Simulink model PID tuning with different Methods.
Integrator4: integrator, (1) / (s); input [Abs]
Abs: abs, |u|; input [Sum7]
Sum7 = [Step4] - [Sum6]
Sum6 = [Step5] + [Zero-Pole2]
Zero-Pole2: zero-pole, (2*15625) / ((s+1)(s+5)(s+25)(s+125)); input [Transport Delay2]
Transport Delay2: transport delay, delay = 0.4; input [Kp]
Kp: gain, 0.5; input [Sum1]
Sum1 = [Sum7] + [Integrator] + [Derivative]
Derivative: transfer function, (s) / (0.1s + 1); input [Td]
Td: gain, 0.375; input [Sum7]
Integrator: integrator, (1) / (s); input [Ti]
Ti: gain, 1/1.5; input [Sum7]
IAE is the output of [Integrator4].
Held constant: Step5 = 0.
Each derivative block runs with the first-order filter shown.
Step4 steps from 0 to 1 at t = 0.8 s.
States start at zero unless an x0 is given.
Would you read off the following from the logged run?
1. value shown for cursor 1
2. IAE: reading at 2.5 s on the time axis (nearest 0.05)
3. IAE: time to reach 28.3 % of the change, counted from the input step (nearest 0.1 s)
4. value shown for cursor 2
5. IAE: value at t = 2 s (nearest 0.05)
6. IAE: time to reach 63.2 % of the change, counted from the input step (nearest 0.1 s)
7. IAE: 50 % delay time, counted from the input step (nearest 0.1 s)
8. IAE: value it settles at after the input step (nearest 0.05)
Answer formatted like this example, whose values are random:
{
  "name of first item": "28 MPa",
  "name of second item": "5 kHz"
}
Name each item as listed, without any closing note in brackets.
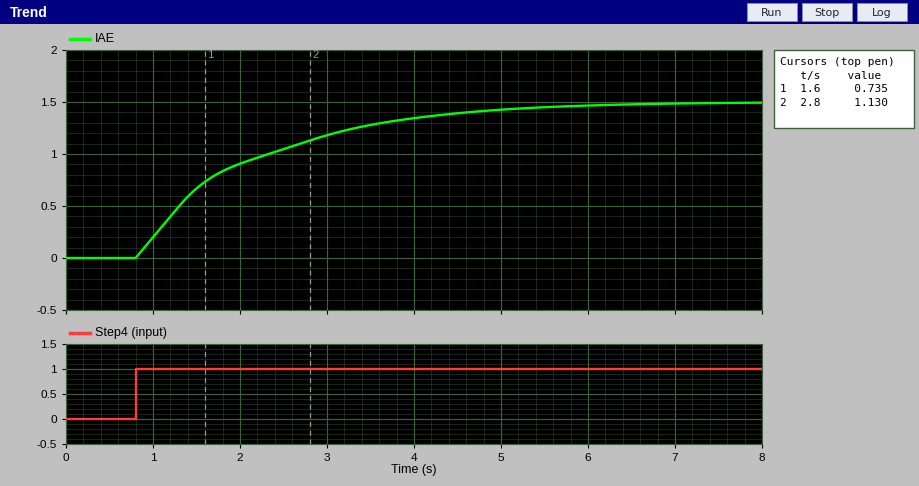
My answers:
{
  "value shown for cursor 1": "0.735",
  "IAE: reading at 2.5 s on the time axis": "1.05",
  "IAE: time to reach 28.3 % of the change, counted from the input step": "0.4 s",
  "value shown for cursor 2": "1.130",
  "IAE: value at t = 2 s": "0.90",
  "IAE: time to reach 63.2 % of the change, counted from the input step": "1.3 s",
  "IAE: 50 % delay time, counted from the input step": "0.8 s",
  "IAE: value it settles at after the input step": "1.50"
}
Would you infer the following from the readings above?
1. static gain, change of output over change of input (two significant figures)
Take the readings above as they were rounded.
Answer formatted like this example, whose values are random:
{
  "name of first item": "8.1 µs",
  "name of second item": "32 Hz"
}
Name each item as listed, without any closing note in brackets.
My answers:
{
  "static gain, change of output over change of input": "1.5"
}
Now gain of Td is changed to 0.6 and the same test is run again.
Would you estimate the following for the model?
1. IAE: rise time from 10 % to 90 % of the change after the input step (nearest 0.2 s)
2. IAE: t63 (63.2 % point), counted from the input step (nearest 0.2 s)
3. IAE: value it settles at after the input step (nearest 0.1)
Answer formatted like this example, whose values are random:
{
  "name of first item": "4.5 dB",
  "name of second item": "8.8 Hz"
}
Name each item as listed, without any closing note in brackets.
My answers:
{
  "IAE: rise time from 10 % to 90 % of the change after the input step": "3.2 s",
  "IAE: t63 (63.2 % point), counted from the input step": "1.6 s",
  "IAE: value it settles at after the input step": "1.5"
}
